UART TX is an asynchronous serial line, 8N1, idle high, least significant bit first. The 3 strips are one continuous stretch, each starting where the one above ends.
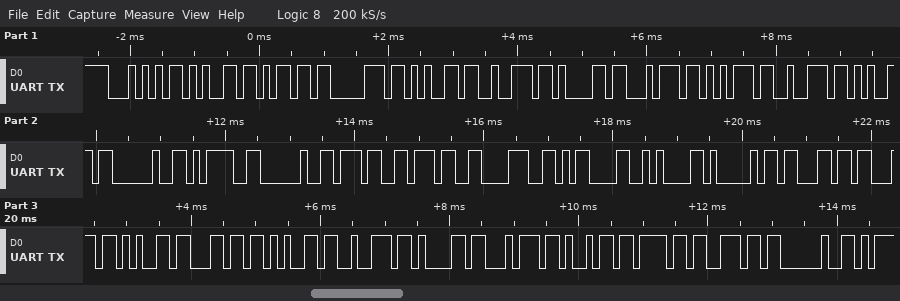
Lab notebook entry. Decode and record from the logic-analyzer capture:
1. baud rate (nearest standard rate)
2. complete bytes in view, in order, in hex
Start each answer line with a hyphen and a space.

- 9600 baud
- 54 65 6D 70 65 72 61 74 75 72 65 20 3D 20 37 37 38 0D 0A 41 63 63 65 6C 65 72 61 74 69 6F 6E 20
